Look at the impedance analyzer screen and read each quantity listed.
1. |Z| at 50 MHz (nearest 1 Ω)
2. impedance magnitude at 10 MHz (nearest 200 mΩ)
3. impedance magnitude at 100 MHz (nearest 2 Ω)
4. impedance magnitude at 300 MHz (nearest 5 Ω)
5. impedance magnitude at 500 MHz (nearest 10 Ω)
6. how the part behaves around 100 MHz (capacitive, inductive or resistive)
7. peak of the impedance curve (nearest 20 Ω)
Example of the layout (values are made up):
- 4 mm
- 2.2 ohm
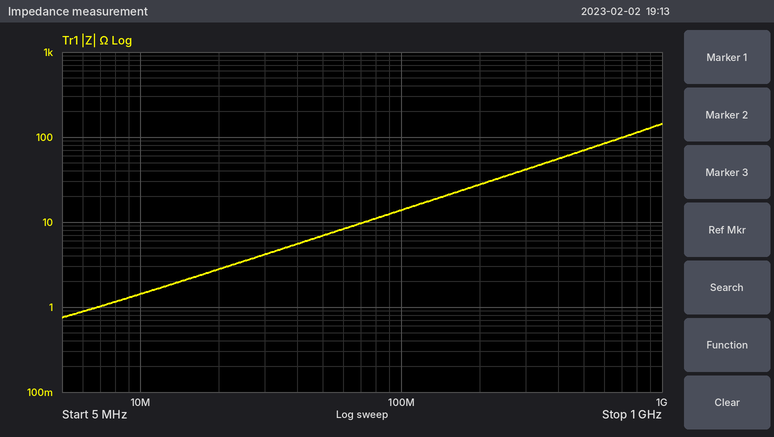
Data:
- 7 Ω
- 1.4 Ω
- 14 Ω
- 40 Ω
- 70 Ω
- inductive
- 140 Ω
